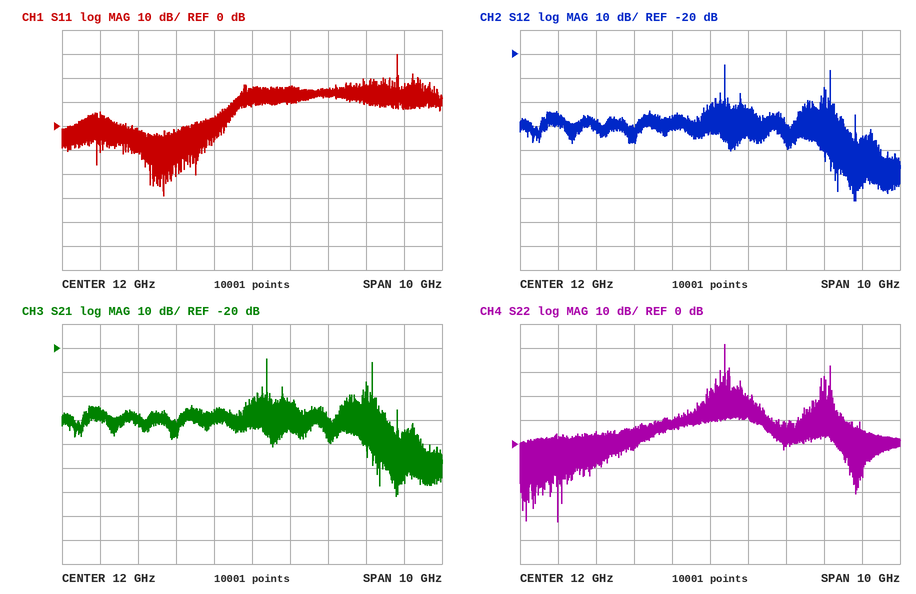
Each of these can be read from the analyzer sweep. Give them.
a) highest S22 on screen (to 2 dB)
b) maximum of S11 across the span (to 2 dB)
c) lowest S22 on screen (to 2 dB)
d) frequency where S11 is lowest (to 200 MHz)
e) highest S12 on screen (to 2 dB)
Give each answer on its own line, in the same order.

42 dB
30 dB
-32 dB
9.6 GHz
-24 dB
